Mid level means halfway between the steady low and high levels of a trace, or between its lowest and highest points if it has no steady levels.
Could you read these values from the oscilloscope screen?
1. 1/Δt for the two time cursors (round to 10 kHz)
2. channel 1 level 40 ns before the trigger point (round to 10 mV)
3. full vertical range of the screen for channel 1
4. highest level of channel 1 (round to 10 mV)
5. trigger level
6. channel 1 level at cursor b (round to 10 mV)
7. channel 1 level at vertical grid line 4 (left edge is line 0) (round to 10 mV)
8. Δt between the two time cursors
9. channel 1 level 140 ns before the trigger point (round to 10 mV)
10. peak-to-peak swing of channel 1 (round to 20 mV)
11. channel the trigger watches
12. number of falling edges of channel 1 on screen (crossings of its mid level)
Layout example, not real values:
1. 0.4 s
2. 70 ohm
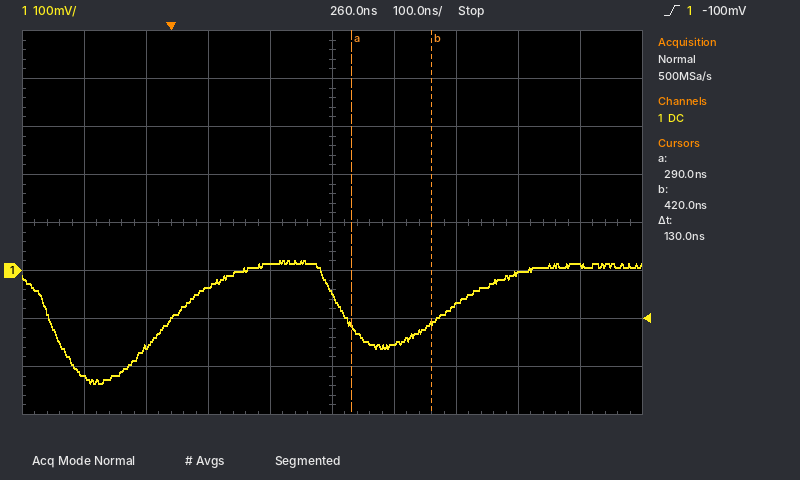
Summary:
1. 7.69 MHz
2. -160 mV
3. 800 mV
4. 20 mV
5. -100 mV
6. -110 mV
7. 10 mV
8. 130 ns
9. -220 mV
10. 260 mV
11. channel 1
12. 2
